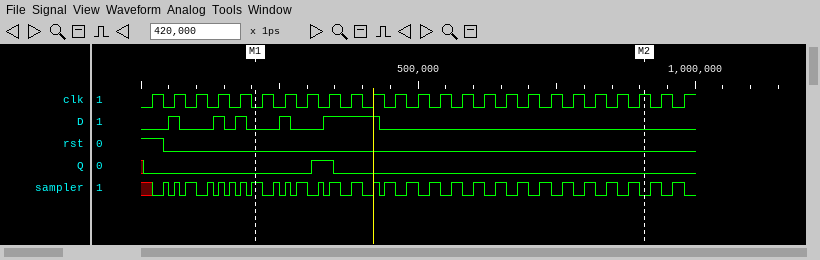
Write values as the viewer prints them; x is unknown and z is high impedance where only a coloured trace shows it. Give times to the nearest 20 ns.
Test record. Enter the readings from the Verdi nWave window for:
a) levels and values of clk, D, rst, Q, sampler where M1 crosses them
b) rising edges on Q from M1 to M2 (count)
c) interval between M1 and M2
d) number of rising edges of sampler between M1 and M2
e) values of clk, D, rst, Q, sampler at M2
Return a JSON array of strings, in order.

["clk=0, D=0, rst=0, Q=0, sampler=1", "1", "700 ns", "19", "clk=1, D=0, rst=0, Q=0, sampler=0"]
